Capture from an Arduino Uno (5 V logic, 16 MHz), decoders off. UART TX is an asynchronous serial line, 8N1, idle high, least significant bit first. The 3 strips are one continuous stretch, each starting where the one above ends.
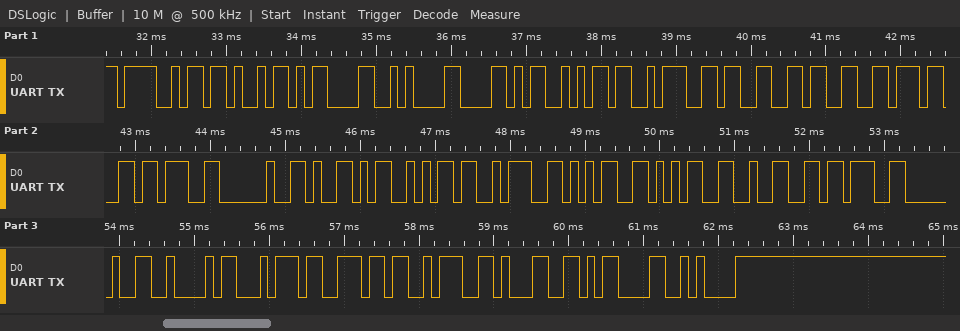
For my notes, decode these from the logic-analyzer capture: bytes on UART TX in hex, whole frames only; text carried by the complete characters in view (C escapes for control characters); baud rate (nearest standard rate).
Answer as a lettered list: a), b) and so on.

a) 4F 4B 0D 0A 58 6A 3A 33 33 37 3B 20 59 6A 3A 35 35 32 3B 20 42 74 6E 3A 31 0D 0A
b) "OK\r\nXj:337; Yj:552; Btn:1\r\n"
c) 9600 baud
